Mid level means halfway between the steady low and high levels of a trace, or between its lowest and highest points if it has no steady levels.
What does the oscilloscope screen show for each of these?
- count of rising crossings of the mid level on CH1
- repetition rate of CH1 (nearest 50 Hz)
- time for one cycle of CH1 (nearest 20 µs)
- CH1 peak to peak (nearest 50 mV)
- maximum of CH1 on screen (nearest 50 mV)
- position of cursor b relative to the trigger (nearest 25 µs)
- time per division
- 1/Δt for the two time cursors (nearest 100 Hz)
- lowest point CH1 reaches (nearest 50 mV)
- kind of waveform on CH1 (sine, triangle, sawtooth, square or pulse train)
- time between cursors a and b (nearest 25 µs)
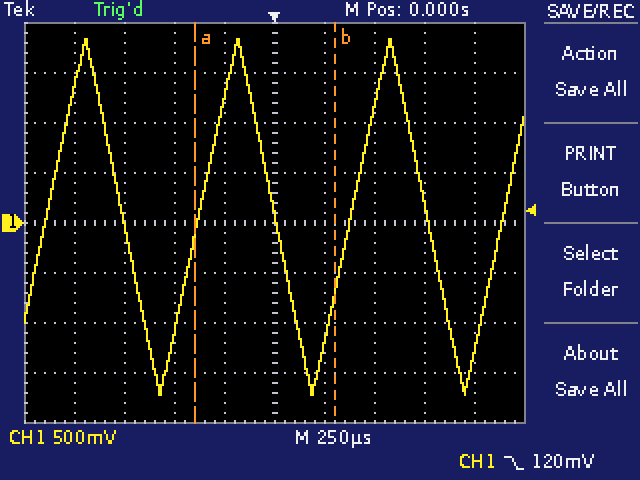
4
1.30 kHz
760 µs
3.55 V
1.85 V
+300 µs
250 µs
1.4 kHz
-1.70 V
triangle
700 µs
